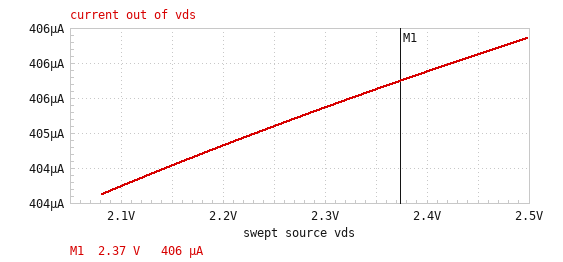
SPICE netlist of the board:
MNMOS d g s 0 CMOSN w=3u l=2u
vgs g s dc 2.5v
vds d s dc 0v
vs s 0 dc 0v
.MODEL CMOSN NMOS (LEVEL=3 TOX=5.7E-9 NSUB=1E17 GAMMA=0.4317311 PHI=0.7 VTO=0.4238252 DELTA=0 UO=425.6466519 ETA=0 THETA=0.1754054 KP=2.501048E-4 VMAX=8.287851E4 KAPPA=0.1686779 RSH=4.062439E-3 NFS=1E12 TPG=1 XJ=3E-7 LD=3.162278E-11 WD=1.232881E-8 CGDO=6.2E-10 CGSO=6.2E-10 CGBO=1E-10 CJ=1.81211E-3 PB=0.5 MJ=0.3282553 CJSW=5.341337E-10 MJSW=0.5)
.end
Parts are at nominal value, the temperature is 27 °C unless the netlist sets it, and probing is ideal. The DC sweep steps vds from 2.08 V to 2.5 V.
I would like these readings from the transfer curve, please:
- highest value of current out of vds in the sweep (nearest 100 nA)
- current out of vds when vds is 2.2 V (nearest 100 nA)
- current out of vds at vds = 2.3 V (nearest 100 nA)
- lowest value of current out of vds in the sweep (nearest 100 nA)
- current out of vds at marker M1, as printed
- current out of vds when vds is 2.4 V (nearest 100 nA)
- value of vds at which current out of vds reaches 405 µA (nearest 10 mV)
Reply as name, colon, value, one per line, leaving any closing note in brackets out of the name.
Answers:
highest value of current out of vds in the sweep: 406.4 µA
current out of vds when vds is 2.2 V: 404.8 µA
current out of vds at vds = 2.3 V: 405.4 µA
lowest value of current out of vds in the sweep: 404.1 µA
current out of vds at marker M1, as printed: 406 µA
current out of vds when vds is 2.4 V: 405.9 µA
value of vds at which current out of vds reaches 405 µA: 2.23 V
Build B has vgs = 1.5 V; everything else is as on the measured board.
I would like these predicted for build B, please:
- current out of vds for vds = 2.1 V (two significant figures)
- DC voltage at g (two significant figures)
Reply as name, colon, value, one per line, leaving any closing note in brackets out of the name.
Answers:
current out of vds for vds = 2.1 V: 140 µA
DC voltage at g: 1.5 V
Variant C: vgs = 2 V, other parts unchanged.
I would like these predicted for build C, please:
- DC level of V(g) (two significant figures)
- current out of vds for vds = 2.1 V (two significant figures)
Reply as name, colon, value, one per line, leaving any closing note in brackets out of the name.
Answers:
DC level of V(g): 2.0 V
current out of vds for vds = 2.1 V: 260 µA
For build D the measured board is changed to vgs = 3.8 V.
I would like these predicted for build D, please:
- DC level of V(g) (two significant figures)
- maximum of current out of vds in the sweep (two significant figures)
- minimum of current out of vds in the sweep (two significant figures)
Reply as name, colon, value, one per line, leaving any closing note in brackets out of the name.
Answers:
DC level of V(g): 3.8 V
maximum of current out of vds in the sweep: 830 µA
minimum of current out of vds in the sweep: 810 µA
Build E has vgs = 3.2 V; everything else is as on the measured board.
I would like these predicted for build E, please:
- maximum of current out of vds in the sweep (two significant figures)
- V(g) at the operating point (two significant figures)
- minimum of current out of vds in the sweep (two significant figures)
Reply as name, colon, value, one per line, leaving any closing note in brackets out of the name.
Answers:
maximum of current out of vds in the sweep: 630 µA
V(g) at the operating point: 3.2 V
minimum of current out of vds in the sweep: 620 µA
